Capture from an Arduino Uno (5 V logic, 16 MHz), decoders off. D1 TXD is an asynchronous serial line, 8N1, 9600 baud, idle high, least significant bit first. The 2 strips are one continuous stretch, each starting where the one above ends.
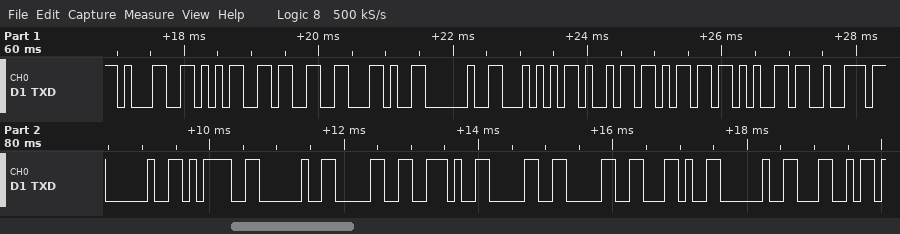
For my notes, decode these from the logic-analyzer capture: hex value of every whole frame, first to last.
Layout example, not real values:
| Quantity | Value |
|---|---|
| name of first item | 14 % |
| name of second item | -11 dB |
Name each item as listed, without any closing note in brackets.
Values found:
| Quantity | Value |
|---|---|
| hex value of every whole frame, first to last | 31 35 33 2C 20 54 69 6D 65 72 20 3D 20 30 2E 30 30 2C 20 4C |
